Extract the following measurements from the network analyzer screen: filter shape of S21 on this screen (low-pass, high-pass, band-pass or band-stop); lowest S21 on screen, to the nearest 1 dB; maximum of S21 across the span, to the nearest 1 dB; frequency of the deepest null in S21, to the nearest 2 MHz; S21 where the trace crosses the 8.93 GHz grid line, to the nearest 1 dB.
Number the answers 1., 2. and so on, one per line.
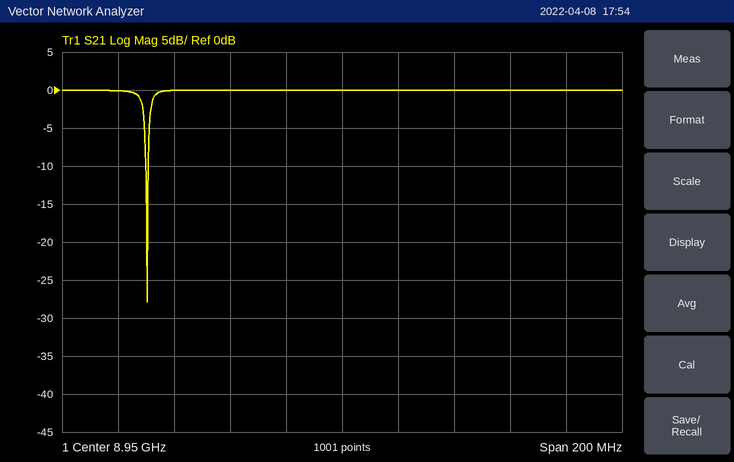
1. band-stop
2. -28 dB
3. 0 dB
4. 8.880 GHz
5. 0 dB
